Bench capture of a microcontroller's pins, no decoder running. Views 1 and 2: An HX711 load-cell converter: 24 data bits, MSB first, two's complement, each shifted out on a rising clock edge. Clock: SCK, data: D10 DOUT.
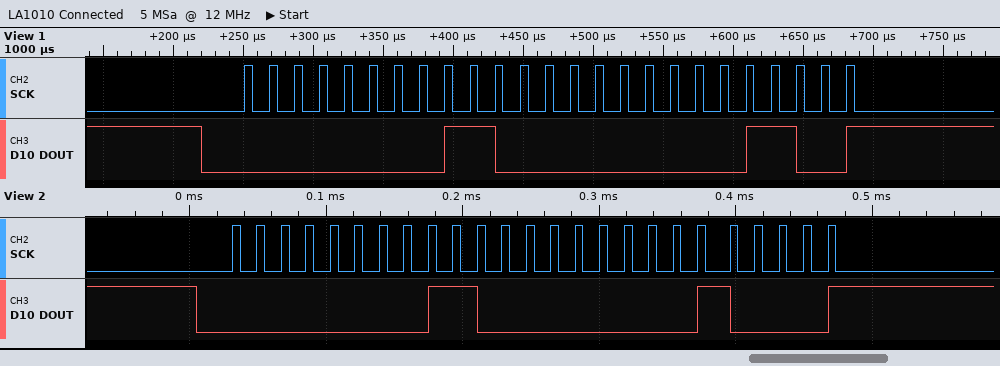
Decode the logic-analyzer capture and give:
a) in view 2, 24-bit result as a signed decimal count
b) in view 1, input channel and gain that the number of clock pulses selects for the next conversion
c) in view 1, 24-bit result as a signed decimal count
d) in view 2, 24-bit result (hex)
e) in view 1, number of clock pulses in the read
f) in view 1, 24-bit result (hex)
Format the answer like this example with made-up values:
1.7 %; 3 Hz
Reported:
49168; channel A, gain 128; 49164; 0x00C010; 25; 0x00C00C
